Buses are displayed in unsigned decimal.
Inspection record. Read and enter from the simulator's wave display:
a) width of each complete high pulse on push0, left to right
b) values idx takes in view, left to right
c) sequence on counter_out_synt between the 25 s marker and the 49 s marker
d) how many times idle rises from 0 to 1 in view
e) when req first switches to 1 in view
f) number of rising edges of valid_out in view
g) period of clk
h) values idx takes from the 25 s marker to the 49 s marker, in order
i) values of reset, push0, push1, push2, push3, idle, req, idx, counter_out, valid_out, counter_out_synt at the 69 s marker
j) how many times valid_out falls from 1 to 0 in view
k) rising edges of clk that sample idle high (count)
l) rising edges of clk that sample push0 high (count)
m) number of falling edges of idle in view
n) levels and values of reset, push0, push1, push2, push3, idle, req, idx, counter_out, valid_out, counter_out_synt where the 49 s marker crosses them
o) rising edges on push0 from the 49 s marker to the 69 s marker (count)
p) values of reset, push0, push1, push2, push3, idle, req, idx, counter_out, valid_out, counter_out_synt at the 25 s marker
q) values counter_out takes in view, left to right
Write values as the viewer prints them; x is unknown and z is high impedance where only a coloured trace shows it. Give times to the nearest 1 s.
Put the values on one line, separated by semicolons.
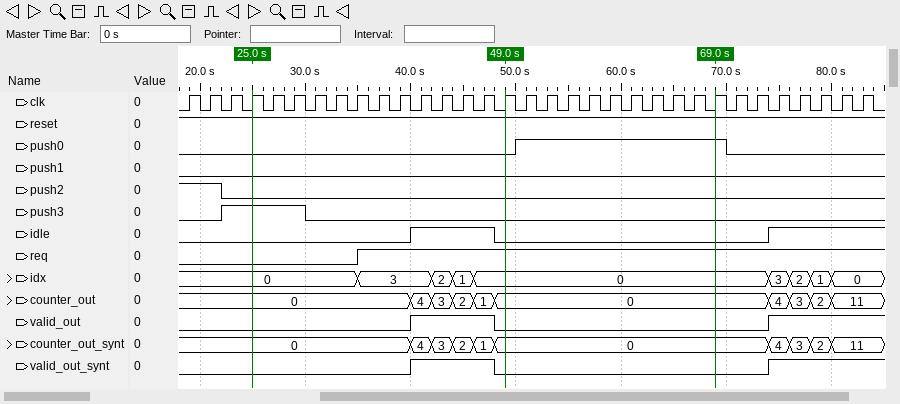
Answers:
20 s; 0, 3, 2, 1, 0, 3, 2, 1, 0; 0, 4, 3, 2, 1, 0; 2; 35 s; 2; 2 s; 0, 3, 2, 1, 0; reset=1, push0=1, push1=0, push2=0, push3=0, idle=0, req=1, idx=0, counter_out=0, valid_out=0, counter_out_synt=0; 1; 9; 10; 1; reset=1, push0=0, push1=0, push2=0, push3=0, idle=0, req=1, idx=0, counter_out=0, valid_out=0, counter_out_synt=0; 1; reset=1, push0=0, push1=0, push2=0, push3=1, idle=0, req=0, idx=0, counter_out=0, valid_out=0, counter_out_synt=0; 0, 4, 3, 2, 1, 0, 4, 3, 2, 11
